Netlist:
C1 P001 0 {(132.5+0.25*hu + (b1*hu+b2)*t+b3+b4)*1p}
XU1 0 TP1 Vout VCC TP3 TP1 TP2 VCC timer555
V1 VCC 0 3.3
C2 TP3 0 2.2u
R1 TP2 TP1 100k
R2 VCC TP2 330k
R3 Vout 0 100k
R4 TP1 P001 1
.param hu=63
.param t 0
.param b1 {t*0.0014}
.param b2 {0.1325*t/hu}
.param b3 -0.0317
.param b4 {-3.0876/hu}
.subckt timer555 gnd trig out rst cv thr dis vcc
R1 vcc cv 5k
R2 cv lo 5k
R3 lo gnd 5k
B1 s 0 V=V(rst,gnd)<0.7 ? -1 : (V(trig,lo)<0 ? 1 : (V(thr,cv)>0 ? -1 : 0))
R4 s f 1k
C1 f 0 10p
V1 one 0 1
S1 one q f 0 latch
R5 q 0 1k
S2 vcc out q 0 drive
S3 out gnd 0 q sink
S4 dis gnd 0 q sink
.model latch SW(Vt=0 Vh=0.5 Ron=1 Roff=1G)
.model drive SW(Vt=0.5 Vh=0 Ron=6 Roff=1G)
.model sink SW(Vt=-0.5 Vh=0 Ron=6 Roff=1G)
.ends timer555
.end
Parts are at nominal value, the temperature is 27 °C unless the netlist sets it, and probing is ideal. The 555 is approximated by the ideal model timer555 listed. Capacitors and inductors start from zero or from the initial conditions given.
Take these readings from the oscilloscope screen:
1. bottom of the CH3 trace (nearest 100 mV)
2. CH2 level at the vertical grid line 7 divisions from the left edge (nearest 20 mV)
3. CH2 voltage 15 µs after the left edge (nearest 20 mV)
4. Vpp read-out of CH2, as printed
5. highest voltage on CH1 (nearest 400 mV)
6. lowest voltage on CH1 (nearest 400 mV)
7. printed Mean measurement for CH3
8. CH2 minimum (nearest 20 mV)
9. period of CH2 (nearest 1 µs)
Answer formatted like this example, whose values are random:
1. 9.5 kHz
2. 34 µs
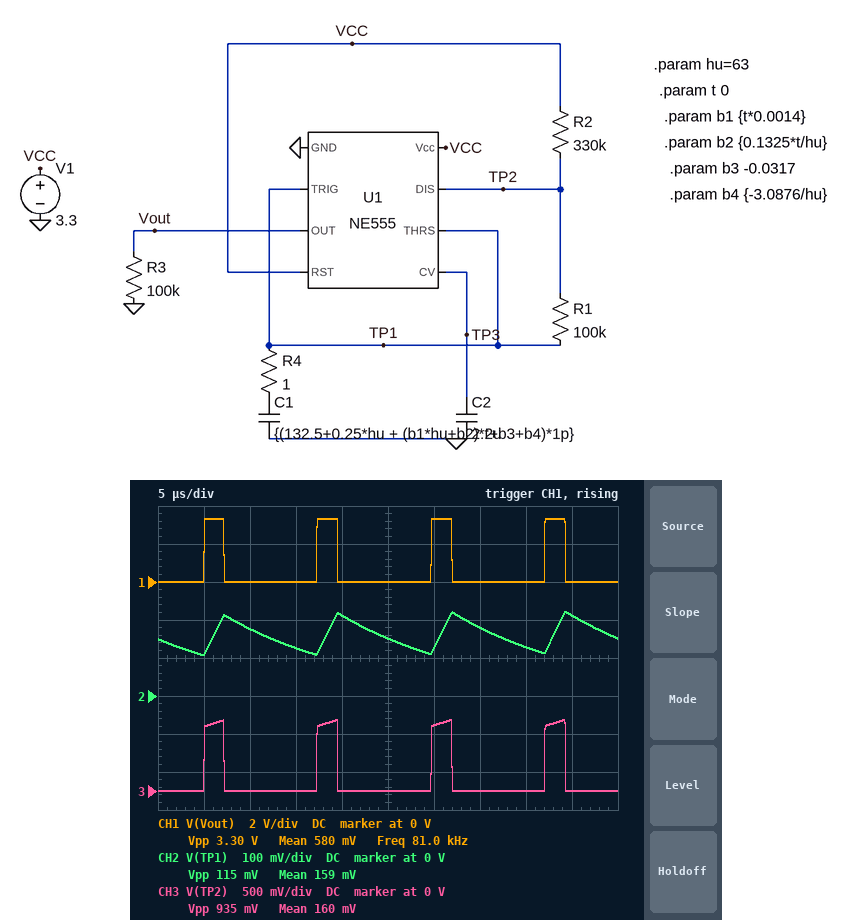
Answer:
1. 0 V
2. 180 mV
3. 120 mV
4. 115 mV
5. 3.2 V
6. 0 V
7. 160 mV
8. 100 mV
9. 12 µs
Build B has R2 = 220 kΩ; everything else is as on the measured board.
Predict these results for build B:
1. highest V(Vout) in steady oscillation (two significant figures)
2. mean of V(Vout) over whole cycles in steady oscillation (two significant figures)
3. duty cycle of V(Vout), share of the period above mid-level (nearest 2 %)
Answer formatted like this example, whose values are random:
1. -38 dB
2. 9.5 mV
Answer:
1. 3.3 V
2. 480 mV
3. 14 %
